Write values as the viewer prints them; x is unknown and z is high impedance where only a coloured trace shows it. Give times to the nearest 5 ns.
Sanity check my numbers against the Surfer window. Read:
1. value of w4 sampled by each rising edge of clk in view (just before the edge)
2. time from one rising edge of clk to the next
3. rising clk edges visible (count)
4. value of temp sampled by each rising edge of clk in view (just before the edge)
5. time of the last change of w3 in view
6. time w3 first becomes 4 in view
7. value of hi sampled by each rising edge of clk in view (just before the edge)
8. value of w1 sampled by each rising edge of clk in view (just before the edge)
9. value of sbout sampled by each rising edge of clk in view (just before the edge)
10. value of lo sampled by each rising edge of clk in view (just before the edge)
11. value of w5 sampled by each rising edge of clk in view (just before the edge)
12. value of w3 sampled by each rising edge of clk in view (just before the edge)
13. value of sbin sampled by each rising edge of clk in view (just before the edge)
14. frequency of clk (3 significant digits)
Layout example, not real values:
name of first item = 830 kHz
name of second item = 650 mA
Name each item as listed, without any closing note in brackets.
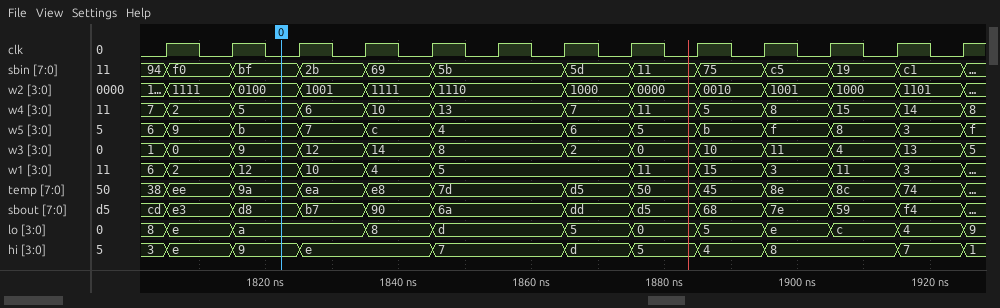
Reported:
value of w4 sampled by each rising edge of clk in view = 7, 2, 5, 6, 10, 13, 13, 7, 11, 5, 8, 15, 14
time from one rising edge of clk to the next = 10 ns
rising clk edges visible = 13
value of temp sampled by each rising edge of clk in view = 38, ee, 9a, ea, e8, 7d, 7d, d5, 50, 45, 8e, 8c, 74
time of the last change of w3 in view = 1925 ns
time w3 first becomes 4 in view = 1905 ns
value of hi sampled by each rising edge of clk in view = 3, e, 9, e, e, 7, 7, d, 5, 4, 8, 8, 7
value of w1 sampled by each rising edge of clk in view = 6, 2, 12, 10, 4, 5, 5, 5, 11, 15, 3, 11, 3
value of sbout sampled by each rising edge of clk in view = cd, e3, d8, b7, 90, 6a, 6a, dd, d5, 68, 7e, 59, f4
value of lo sampled by each rising edge of clk in view = 8, e, a, a, 8, d, d, 5, 0, 5, e, c, 4
value of w5 sampled by each rising edge of clk in view = 6, 9, b, 7, c, 4, 4, 6, 5, b, f, 8, 3
value of w3 sampled by each rising edge of clk in view = 1, 0, 9, 12, 14, 8, 8, 2, 0, 10, 11, 4, 13
value of sbin sampled by each rising edge of clk in view = 94, f0, bf, 2b, 69, 5b, 5b, 5d, 11, 75, c5, 19, c1
frequency of clk = 100 MHz
